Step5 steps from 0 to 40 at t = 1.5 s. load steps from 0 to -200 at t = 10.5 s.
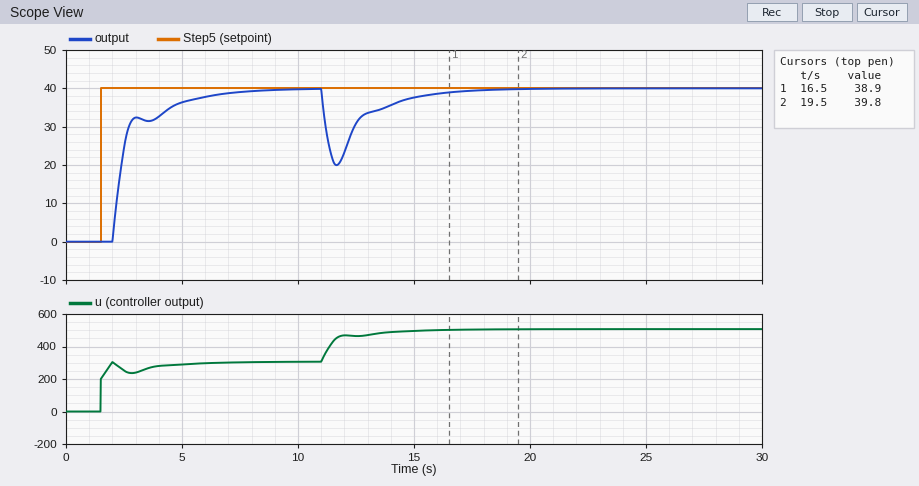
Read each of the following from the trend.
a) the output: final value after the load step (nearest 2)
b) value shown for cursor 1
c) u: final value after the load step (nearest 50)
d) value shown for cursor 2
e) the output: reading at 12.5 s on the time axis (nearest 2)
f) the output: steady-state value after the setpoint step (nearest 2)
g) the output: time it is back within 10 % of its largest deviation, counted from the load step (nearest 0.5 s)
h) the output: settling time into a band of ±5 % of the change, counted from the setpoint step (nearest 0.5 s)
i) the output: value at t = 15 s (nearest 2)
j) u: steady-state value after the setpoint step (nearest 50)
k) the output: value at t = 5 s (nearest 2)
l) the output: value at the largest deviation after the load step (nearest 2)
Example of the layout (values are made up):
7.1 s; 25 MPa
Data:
40; 38.9; 500; 39.8; 30; 40; 5.0 s; 4.5 s; 38; 300; 36; 20
